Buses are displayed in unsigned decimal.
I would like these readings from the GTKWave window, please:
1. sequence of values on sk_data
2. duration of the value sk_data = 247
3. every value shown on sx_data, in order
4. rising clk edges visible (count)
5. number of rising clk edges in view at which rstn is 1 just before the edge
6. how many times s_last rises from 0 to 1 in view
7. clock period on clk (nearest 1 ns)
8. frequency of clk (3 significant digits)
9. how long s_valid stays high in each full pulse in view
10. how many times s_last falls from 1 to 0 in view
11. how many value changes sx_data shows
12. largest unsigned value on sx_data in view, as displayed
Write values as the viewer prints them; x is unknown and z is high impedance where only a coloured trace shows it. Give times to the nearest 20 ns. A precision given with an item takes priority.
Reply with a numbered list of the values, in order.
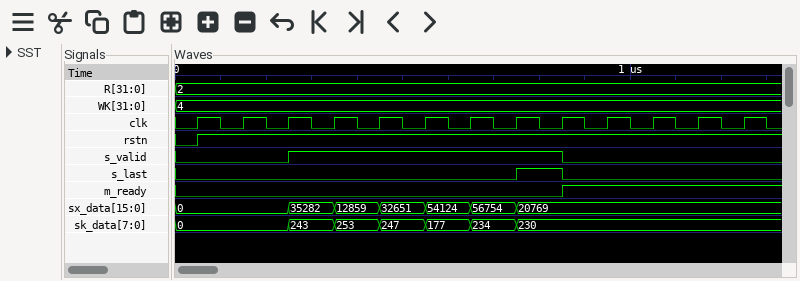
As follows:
1. 0, 243, 253, 247, 177, 234, 230
2. 100 ns
3. 0, 35282, 12859, 32651, 54124, 56754, 20769
4. 13
5. 12
6. 1
7. 100 ns
8. 10.0 MHz
9. 600 ns
10. 1
11. 6
12. 56754
